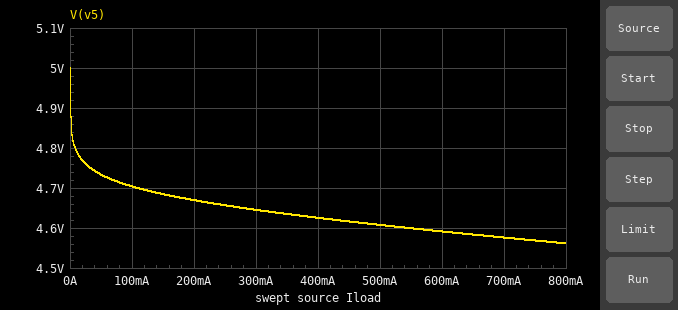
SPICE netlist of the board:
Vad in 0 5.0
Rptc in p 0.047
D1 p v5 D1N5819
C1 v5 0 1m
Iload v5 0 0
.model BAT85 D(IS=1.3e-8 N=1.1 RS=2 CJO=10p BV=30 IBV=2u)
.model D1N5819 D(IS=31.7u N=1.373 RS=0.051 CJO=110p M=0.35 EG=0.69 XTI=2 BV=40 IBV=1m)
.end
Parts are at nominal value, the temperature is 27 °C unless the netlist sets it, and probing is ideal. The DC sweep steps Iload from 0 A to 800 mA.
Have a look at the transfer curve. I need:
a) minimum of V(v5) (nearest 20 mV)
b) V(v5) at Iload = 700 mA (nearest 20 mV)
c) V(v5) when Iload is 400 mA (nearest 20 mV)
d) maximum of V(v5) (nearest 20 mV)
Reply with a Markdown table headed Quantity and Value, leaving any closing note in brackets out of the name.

| Quantity | Value |
|---|---|
| minimum of V(v5) | 4.56 V |
| V(v5) at Iload = 700 mA | 4.58 V |
| V(v5) when Iload is 400 mA | 4.62 V |
| maximum of V(v5) | 5.00 V |
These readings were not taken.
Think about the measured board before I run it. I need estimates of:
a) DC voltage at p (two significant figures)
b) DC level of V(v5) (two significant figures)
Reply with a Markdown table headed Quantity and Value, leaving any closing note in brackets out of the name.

| Quantity | Value |
|---|---|
| DC voltage at p | 5.0 V |
| DC level of V(v5) | 5.0 V |
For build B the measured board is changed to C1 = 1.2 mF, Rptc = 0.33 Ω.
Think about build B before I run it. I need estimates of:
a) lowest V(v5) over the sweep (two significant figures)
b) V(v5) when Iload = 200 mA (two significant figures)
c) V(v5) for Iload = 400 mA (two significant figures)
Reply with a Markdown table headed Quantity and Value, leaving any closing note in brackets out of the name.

| Quantity | Value |
|---|---|
| lowest V(v5) over the sweep | 4.3 V |
| V(v5) when Iload = 200 mA | 4.6 V |
| V(v5) for Iload = 400 mA | 4.5 V |
